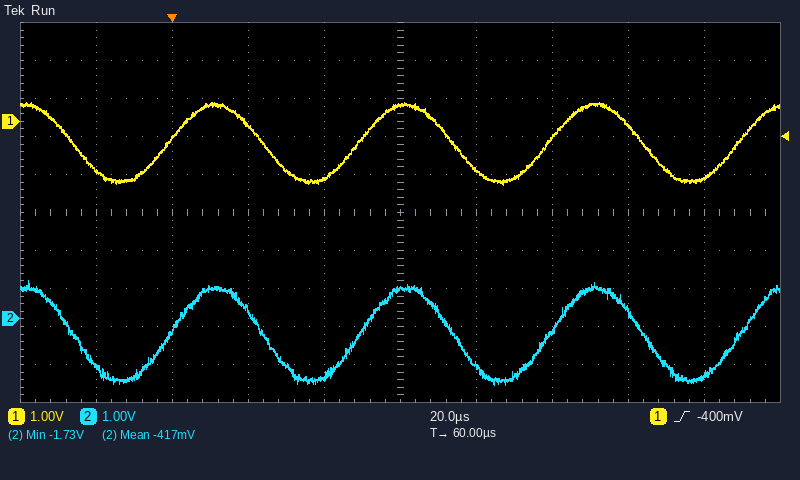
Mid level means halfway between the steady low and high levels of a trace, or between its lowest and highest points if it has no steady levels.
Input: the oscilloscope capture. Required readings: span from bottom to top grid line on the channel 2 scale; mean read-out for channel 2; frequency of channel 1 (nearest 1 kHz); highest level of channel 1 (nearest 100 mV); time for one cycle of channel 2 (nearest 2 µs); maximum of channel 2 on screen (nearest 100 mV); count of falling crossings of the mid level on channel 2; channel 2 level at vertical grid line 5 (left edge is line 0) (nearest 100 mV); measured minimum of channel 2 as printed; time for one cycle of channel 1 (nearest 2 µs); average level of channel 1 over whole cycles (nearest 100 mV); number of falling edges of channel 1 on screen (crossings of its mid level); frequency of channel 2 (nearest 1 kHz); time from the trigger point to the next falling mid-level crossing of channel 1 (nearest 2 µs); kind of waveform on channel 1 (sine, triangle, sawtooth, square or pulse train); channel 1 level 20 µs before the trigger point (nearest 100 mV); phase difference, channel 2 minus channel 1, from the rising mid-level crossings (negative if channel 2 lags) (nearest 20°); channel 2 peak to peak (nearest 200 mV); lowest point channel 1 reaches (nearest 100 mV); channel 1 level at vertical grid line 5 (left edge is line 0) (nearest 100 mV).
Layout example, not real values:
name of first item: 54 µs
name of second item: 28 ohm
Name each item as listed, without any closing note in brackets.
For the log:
span from bottom to top grid line on the channel 2 scale: 10 V
mean read-out for channel 2: -417 mV
frequency of channel 1: 20 kHz
highest level of channel 1: 500 mV
time for one cycle of channel 2: 50 µs
maximum of channel 2 on screen: 1.0 V
count of falling crossings of the mid level on channel 2: 4
channel 2 level at vertical grid line 5 (left edge is line 0): 800 mV
measured minimum of channel 2 as printed: -1.73 V
time for one cycle of channel 1: 50 µs
average level of channel 1 over whole cycles: -600 mV
number of falling edges of channel 1 on screen: 4
frequency of channel 2: 20 kHz
time from the trigger point to the next falling mid-level crossing of channel 1: 24 µs
kind of waveform on channel 1: sine
channel 1 level 20 µs before the trigger point: -1.3 V
phase difference, channel 2 minus channel 1, from the rising mid-level crossings (negative if channel 2 lags): 0°
channel 2 peak to peak: 2.8 V
lowest point channel 1 reaches: -1.7 V
channel 1 level at vertical grid line 5 (left edge is line 0): 400 mV
